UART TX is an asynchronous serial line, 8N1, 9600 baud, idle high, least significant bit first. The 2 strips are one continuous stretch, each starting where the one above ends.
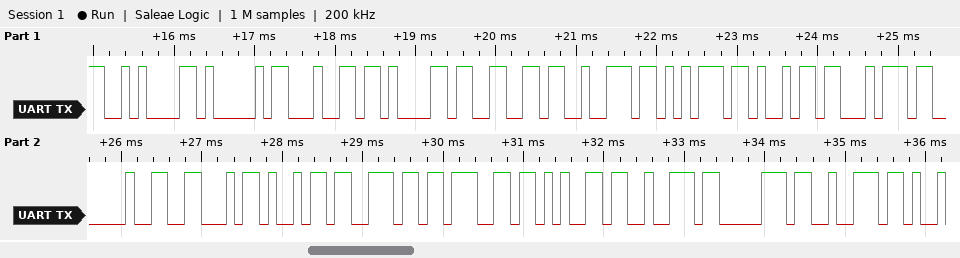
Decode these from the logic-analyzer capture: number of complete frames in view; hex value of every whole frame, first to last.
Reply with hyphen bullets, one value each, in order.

- 18
- 0A 41 64 61 66 72 75 69 74 20 46 69 6E 67 65 72 70 72
